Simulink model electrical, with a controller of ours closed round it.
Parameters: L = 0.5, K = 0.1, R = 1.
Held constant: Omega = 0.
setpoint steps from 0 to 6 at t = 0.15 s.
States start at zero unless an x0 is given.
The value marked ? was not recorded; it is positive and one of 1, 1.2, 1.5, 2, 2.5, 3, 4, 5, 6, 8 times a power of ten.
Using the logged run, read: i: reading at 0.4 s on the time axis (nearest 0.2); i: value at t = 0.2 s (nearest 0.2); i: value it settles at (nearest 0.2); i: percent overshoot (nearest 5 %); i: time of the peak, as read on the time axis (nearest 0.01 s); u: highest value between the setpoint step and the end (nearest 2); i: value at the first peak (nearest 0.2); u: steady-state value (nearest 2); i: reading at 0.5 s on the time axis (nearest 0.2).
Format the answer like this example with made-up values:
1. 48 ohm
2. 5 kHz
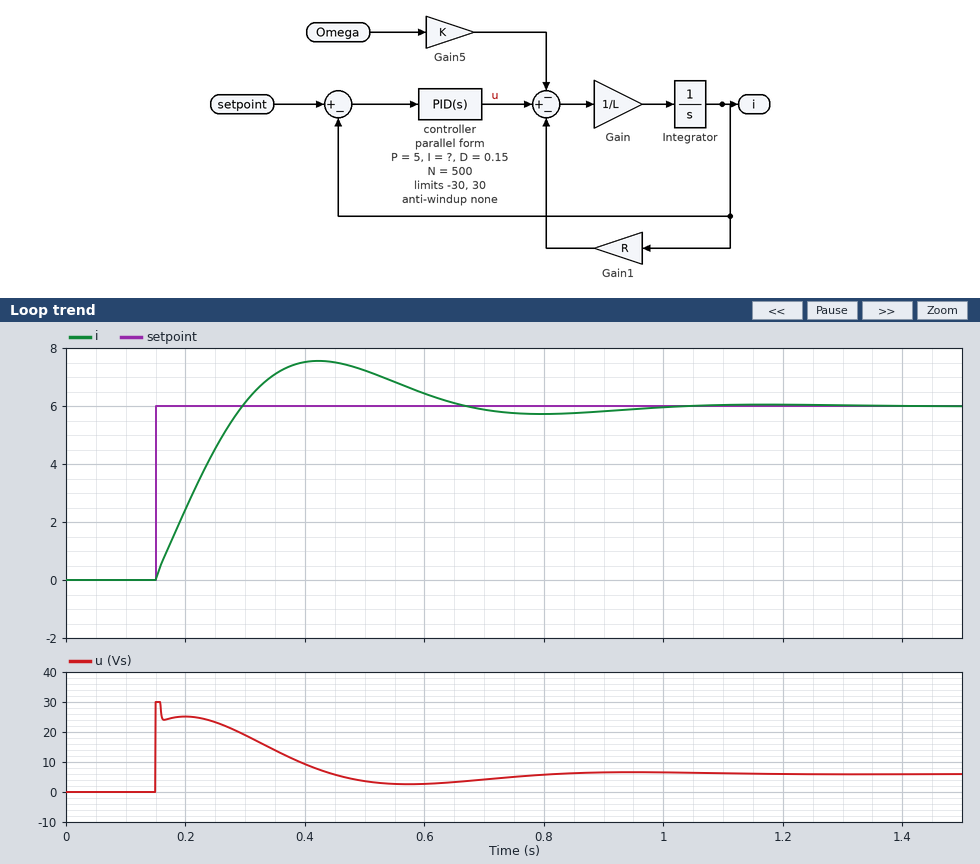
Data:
1. 7.6
2. 2.4
3. 6.0
4. 25 %
5. 0.42 s
6. 30
7. 7.6
8. 6
9. 7.2
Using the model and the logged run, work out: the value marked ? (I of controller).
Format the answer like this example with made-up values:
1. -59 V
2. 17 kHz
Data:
1. 60
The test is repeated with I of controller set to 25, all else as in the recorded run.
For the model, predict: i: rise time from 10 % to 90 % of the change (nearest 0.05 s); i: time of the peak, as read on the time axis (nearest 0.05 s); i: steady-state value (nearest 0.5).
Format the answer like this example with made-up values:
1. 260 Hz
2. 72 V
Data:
1. 0.15 s
2. 0.55 s
3. 6.0
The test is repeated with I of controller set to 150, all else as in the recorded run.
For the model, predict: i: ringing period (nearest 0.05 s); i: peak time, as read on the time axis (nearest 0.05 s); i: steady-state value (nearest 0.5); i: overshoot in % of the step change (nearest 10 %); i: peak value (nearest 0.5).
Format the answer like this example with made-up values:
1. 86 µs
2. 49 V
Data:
1. 0.45 s
2. 0.35 s
3. 6.0
4. 50 %
5. 9.0
